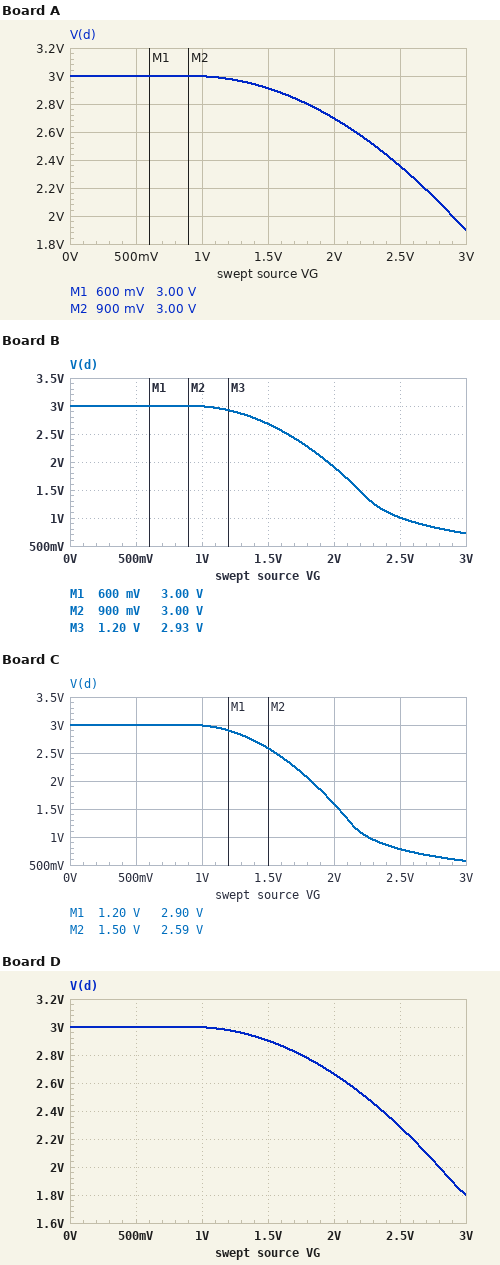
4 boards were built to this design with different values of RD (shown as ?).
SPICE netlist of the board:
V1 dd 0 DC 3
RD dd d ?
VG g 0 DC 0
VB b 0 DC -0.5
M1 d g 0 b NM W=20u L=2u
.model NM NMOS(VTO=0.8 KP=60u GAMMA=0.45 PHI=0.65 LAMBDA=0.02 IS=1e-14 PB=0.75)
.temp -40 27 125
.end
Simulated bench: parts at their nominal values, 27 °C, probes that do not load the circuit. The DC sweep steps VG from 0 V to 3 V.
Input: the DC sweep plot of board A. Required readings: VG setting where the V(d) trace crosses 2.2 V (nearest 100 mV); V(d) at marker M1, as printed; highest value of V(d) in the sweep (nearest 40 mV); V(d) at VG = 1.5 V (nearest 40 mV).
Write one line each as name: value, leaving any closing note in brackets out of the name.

VG setting where the V(d) trace crosses 2.2 V: 2.7 V
V(d) at marker M1, as printed: 3.00 V
highest value of V(d) in the sweep: 3.00 V
V(d) at VG = 1.5 V: 2.92 V
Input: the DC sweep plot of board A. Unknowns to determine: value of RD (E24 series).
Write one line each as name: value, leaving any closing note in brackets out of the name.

value of RD: 820 Ω
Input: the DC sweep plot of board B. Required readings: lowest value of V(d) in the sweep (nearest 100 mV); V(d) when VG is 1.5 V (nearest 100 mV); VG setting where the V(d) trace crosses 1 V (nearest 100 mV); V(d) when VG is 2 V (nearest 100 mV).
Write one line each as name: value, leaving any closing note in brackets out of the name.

lowest value of V(d) in the sweep: 700 mV
V(d) when VG is 1.5 V: 2.7 V
VG setting where the V(d) trace crosses 1 V: 2.5 V
V(d) when VG is 2 V: 1.9 V
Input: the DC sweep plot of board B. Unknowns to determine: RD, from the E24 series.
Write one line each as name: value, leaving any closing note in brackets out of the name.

RD, from the E24 series: 3 kΩ
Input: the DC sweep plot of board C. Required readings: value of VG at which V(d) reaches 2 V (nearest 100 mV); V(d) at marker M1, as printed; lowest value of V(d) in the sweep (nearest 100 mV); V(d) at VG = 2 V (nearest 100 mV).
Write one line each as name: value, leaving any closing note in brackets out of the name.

value of VG at which V(d) reaches 2 V: 1.8 V
V(d) at marker M1, as printed: 2.90 V
lowest value of V(d) in the sweep: 600 mV
V(d) at VG = 2 V: 1.6 V
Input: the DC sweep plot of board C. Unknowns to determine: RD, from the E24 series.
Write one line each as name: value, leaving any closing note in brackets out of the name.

RD, from the E24 series: 3.9 kΩ
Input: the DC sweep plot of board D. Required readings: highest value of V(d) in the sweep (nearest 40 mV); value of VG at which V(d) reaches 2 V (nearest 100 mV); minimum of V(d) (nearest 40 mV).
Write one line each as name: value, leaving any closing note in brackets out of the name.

highest value of V(d) in the sweep: 3.00 V
value of VG at which V(d) reaches 2 V: 2.8 V
minimum of V(d): 1.80 V
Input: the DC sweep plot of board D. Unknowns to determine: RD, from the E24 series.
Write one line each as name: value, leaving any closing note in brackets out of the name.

RD, from the E24 series: 910 Ω
